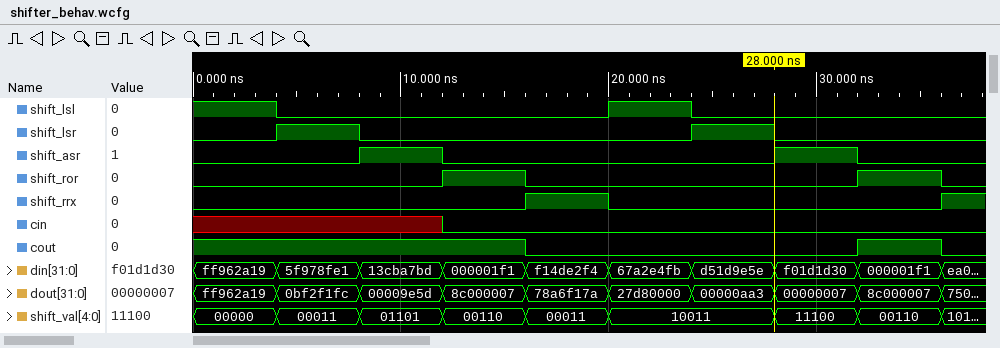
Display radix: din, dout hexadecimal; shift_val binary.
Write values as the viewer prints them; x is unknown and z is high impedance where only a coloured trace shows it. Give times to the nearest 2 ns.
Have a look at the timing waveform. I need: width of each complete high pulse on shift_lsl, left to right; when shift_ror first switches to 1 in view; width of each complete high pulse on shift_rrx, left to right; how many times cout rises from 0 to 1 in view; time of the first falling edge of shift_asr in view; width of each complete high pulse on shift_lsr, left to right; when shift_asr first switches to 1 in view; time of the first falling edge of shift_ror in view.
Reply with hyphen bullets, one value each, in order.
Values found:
- 4 ns
- 12 ns
- 4 ns
- 1
- 12 ns
- 4 ns, 4 ns
- 8 ns
- 16 ns
